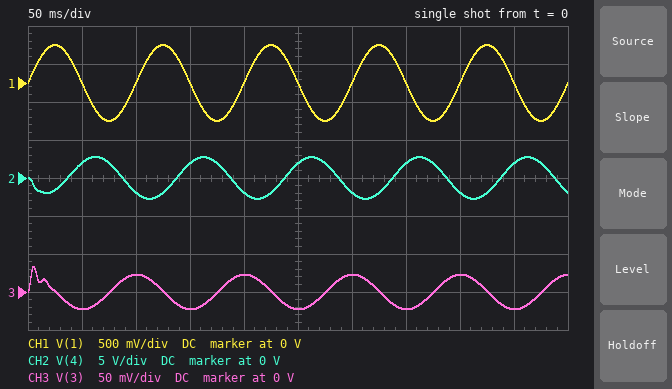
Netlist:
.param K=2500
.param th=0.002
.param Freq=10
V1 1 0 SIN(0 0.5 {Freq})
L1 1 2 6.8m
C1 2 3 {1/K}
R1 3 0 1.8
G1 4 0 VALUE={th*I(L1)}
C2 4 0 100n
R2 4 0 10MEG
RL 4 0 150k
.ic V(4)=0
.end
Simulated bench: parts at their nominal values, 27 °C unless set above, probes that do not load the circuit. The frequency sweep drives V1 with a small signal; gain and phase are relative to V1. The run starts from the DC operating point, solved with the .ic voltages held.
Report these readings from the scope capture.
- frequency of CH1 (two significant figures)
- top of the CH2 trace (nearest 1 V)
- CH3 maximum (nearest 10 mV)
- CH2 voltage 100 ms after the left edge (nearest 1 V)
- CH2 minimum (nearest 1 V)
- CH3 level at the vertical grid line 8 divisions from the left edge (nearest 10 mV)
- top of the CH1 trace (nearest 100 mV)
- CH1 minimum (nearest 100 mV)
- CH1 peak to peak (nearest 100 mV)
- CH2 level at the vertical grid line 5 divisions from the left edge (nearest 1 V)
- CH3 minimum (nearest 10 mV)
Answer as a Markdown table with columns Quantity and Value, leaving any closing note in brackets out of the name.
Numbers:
| Quantity | Value |
|---|---|
| frequency of CH1 | 10 Hz |
| top of the CH2 trace | 3 V |
| CH3 maximum | 30 mV |
| CH2 voltage 100 ms after the left edge | -2 V |
| CH2 minimum | -3 V |
| CH3 level at the vertical grid line 8 divisions from the left edge | 20 mV |
| top of the CH1 trace | 500 mV |
| CH1 minimum | -500 mV |
| CH1 peak to peak | 1.0 V |
| CH2 level at the vertical grid line 5 divisions from the left edge | 2 V |
| CH3 minimum | -20 mV |
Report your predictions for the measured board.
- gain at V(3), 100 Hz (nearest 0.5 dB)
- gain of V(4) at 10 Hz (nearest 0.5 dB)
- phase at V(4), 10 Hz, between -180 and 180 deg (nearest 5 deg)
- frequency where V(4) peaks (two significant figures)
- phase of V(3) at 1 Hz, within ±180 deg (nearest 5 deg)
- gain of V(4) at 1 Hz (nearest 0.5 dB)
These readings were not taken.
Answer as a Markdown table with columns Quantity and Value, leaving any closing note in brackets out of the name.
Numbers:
| Quantity | Value |
|---|---|
| gain at V(3), 100 Hz | 0 dB |
| gain of V(4) at 10 Hz | 15.0 dB |
| phase at V(4), 10 Hz, between -180 and 180 deg | -135 deg |
| frequency where V(4) peaks | 92 Hz |
| phase of V(3) at 1 Hz, within ±180 deg | 90 deg |
| gain of V(4) at 1 Hz | -2.5 dB |
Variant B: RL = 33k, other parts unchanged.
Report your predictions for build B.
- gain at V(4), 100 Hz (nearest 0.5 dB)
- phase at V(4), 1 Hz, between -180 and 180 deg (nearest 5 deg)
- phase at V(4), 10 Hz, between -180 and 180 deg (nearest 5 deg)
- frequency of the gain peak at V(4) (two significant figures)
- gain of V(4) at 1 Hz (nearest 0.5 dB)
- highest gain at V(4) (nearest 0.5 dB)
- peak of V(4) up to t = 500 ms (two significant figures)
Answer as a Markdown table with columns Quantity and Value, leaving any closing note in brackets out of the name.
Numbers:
| Quantity | Value |
|---|---|
| gain at V(4), 100 Hz | 24.0 dB |
| phase at V(4), 1 Hz, between -180 and 180 deg | -90 deg |
| phase at V(4), 10 Hz, between -180 and 180 deg | -105 deg |
| frequency of the gain peak at V(4) | 93 Hz |
| gain of V(4) at 1 Hz | -15.5 dB |
| highest gain at V(4) | 24.5 dB |
| peak of V(4) up to t = 500 ms | 820 mV |
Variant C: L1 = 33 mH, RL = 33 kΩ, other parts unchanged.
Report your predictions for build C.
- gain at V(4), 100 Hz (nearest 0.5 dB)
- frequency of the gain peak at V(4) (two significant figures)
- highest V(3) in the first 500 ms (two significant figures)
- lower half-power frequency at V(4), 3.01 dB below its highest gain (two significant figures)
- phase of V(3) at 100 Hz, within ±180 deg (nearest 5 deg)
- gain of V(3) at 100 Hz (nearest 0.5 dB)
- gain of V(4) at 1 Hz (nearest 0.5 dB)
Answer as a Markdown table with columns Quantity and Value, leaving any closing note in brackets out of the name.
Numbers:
| Quantity | Value |
|---|---|
| gain at V(4), 100 Hz | 4.5 dB |
| frequency of the gain peak at V(4) | 44 Hz |
| highest V(3) in the first 500 ms | 36 mV |
| lower half-power frequency at V(4), 3.01 dB below its highest gain | 39 Hz |
| phase of V(3) at 100 Hz, within ±180 deg | -85 deg |
| gain of V(3) at 100 Hz | -19.5 dB |
| gain of V(4) at 1 Hz | -15.5 dB |
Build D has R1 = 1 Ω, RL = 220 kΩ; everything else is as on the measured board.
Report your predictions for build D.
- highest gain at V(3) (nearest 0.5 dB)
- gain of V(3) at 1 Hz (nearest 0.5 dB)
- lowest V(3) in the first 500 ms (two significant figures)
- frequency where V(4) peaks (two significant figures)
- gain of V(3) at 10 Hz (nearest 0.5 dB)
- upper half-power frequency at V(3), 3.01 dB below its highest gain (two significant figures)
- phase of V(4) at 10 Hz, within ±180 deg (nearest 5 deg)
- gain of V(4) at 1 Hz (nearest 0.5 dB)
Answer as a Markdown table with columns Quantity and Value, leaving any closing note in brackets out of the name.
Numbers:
| Quantity | Value |
|---|---|
| highest gain at V(3) | 0 dB |
| gain of V(3) at 1 Hz | -52.0 dB |
| lowest V(3) in the first 500 ms | -13 mV |
| frequency where V(4) peaks | 95 Hz |
| gain of V(3) at 10 Hz | -32.0 dB |
| upper half-power frequency at V(3), 3.01 dB below its highest gain | 110 Hz |
| phase of V(4) at 10 Hz, within ±180 deg | -145 deg |
| gain of V(4) at 1 Hz | 0.5 dB |
